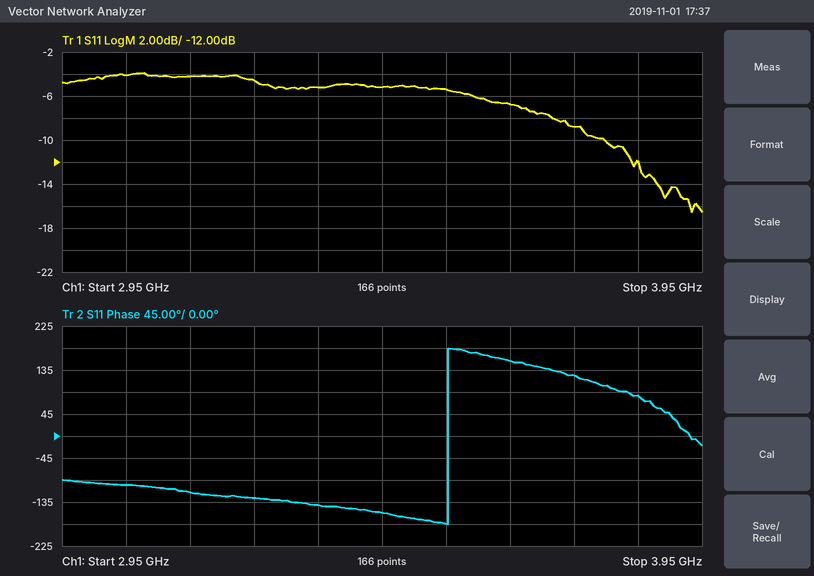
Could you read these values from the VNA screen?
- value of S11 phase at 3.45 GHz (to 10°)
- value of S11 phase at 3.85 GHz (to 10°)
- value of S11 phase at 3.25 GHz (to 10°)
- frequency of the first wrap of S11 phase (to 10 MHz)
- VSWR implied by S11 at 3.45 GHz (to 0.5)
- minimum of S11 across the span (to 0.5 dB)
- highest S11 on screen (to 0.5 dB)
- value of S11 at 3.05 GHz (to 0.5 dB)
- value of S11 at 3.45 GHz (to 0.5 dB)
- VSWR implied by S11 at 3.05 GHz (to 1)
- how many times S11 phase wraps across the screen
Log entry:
-160°
80°
-130°
3.55 GHz
3.5
-16.5 dB
-4.0 dB
-4.0 dB
-5.0 dB
4
1
